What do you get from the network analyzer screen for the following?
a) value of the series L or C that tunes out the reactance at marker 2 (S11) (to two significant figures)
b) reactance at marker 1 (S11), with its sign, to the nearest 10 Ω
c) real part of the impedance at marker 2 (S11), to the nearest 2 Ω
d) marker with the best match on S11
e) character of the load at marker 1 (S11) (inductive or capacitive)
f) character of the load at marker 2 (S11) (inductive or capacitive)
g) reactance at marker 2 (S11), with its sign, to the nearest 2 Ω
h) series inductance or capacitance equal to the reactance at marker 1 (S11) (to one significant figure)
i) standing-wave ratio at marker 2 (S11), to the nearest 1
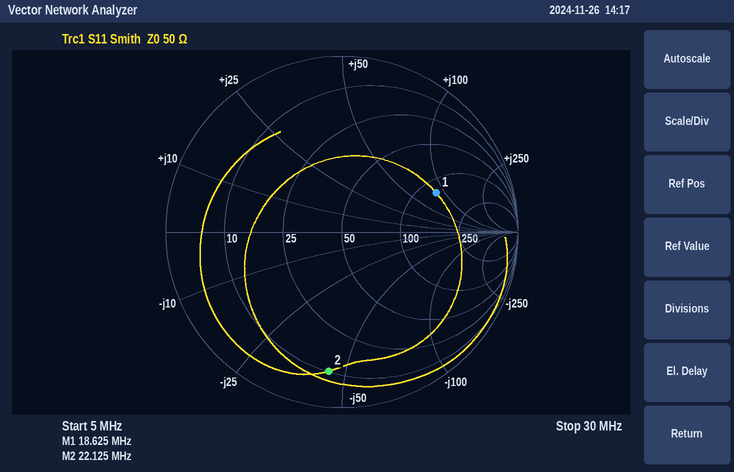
320 nH
+80 Ω
10 Ω
marker 1
inductive
capacitive
-44 Ω
700 nH
9
